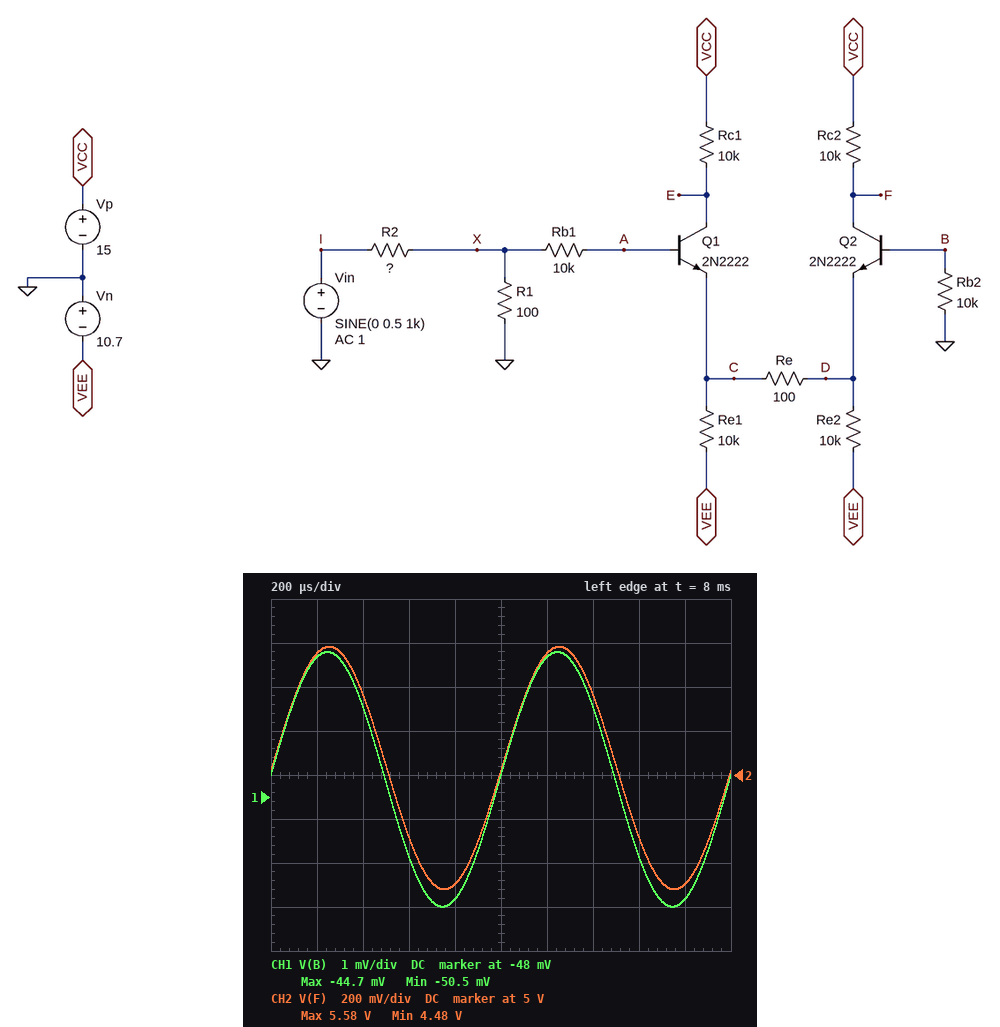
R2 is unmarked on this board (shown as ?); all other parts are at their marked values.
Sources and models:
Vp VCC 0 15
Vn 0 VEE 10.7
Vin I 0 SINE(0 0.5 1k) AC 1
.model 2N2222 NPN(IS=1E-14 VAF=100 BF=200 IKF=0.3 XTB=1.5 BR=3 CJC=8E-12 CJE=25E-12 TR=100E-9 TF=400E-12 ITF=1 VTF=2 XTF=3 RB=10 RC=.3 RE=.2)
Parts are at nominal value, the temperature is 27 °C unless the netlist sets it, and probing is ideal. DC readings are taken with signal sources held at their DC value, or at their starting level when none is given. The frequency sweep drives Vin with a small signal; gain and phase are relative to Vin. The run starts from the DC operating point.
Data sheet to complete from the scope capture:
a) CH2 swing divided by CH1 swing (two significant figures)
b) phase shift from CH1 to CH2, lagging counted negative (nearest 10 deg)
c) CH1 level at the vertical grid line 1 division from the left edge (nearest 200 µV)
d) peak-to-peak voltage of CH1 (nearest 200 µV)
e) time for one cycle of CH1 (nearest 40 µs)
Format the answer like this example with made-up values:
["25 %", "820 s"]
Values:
["190", "0 deg", "-44.8 mV", "5.8 mV", "1.00 ms"]
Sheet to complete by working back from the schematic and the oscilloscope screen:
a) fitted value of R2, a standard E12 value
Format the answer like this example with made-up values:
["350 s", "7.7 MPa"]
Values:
["3.3 kΩ"]
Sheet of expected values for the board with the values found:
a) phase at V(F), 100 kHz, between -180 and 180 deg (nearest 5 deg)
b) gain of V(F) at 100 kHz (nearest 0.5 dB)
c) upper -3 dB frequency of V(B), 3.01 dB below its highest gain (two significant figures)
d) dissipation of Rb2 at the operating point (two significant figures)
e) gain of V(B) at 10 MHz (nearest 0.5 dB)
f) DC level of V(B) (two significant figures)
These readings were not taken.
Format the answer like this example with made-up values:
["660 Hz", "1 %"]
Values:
["-65 deg", "-6.5 dB", "1.6 MHz", "230 nW", "-46.0 dB", "-48 mV"]
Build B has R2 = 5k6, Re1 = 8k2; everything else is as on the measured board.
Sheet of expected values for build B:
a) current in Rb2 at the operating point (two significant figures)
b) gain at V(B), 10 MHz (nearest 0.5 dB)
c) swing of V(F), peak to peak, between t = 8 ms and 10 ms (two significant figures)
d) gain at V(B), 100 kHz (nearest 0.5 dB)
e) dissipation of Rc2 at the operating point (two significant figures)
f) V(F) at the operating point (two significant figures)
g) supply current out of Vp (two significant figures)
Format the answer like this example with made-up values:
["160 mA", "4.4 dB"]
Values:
["5.1 µA", "-51.0 dB", "660 mV", "-42.5 dB", "11 mW", "4.4 V", "2.2 mA"]
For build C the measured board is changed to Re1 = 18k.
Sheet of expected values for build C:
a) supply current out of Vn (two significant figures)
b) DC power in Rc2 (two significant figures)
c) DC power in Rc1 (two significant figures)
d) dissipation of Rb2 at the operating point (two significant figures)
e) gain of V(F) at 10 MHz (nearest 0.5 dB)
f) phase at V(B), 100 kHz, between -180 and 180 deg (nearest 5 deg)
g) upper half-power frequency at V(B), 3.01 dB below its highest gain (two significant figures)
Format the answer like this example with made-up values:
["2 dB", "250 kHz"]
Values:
["1.6 mA", "7.4 mW", "4.8 mW", "160 nW", "-45.0 dB", "15 deg", "1.9 MHz"]
